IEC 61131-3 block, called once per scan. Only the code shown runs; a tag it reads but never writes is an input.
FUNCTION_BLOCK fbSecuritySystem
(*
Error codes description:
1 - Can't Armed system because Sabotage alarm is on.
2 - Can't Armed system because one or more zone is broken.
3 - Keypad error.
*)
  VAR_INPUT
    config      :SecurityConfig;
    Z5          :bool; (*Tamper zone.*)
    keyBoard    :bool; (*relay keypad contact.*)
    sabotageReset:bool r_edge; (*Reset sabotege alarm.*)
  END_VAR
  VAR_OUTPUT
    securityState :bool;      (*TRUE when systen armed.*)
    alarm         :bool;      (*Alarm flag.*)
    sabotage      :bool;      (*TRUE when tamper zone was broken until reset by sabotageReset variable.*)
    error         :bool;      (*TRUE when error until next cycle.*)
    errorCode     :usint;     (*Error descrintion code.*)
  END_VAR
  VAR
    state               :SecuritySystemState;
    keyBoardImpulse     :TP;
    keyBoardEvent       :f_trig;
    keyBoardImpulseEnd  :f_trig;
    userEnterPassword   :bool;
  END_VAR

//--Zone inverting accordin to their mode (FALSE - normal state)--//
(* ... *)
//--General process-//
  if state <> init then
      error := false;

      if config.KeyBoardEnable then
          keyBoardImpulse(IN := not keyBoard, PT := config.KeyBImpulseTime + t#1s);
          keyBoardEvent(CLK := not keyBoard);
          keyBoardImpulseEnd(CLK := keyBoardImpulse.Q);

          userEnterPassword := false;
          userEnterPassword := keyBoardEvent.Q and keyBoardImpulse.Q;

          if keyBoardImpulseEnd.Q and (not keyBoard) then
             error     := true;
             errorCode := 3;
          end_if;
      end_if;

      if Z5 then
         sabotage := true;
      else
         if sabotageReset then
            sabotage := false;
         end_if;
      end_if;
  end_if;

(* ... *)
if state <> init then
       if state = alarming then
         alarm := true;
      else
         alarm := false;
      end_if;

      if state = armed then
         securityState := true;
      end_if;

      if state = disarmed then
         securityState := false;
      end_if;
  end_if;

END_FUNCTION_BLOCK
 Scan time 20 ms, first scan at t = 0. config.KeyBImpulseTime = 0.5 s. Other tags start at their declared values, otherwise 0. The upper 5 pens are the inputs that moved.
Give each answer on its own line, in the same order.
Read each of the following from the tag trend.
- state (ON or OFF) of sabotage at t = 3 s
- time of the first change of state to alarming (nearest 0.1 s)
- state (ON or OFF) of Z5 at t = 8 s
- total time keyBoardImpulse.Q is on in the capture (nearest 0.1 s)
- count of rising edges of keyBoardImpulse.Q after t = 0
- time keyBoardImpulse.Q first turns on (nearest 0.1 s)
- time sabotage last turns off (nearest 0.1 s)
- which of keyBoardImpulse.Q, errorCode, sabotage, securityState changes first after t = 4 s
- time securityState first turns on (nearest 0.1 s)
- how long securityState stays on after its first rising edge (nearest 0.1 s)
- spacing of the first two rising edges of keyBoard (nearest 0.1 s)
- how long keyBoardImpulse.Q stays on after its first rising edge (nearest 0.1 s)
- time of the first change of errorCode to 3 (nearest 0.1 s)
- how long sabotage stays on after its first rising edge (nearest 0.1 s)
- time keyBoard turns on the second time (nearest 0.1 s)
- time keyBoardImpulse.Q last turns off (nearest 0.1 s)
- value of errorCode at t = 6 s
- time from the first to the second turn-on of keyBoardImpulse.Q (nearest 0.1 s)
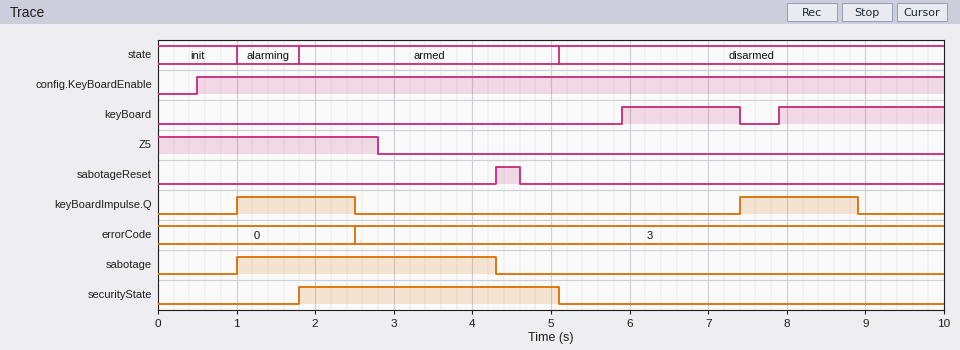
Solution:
ON
1.0 s
OFF
3.0 s
2
1.0 s
4.3 s
sabotage
1.8 s
3.3 s
2.0 s
1.5 s
2.5 s
3.3 s
7.9 s
8.9 s
3
6.4 s
